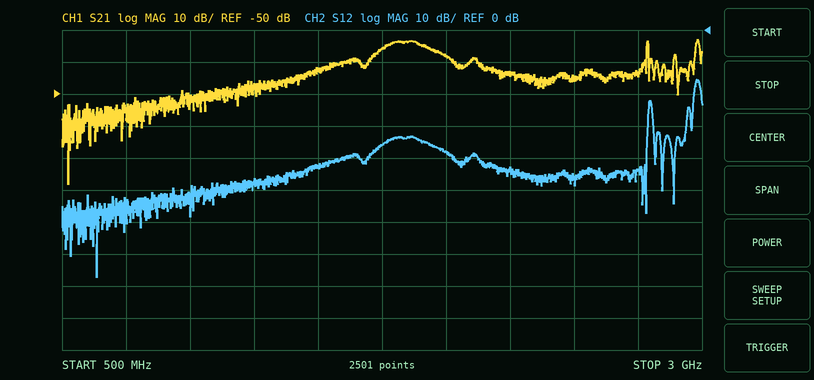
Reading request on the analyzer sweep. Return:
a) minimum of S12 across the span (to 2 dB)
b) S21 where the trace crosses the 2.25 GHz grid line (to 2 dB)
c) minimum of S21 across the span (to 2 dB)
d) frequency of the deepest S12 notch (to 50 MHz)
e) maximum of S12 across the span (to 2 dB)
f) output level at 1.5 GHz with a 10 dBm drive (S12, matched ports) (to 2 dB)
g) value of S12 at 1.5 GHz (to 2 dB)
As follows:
-78 dB
-44 dB
-78 dB
650 MHz
-16 dB
-32 dBm
-42 dB
